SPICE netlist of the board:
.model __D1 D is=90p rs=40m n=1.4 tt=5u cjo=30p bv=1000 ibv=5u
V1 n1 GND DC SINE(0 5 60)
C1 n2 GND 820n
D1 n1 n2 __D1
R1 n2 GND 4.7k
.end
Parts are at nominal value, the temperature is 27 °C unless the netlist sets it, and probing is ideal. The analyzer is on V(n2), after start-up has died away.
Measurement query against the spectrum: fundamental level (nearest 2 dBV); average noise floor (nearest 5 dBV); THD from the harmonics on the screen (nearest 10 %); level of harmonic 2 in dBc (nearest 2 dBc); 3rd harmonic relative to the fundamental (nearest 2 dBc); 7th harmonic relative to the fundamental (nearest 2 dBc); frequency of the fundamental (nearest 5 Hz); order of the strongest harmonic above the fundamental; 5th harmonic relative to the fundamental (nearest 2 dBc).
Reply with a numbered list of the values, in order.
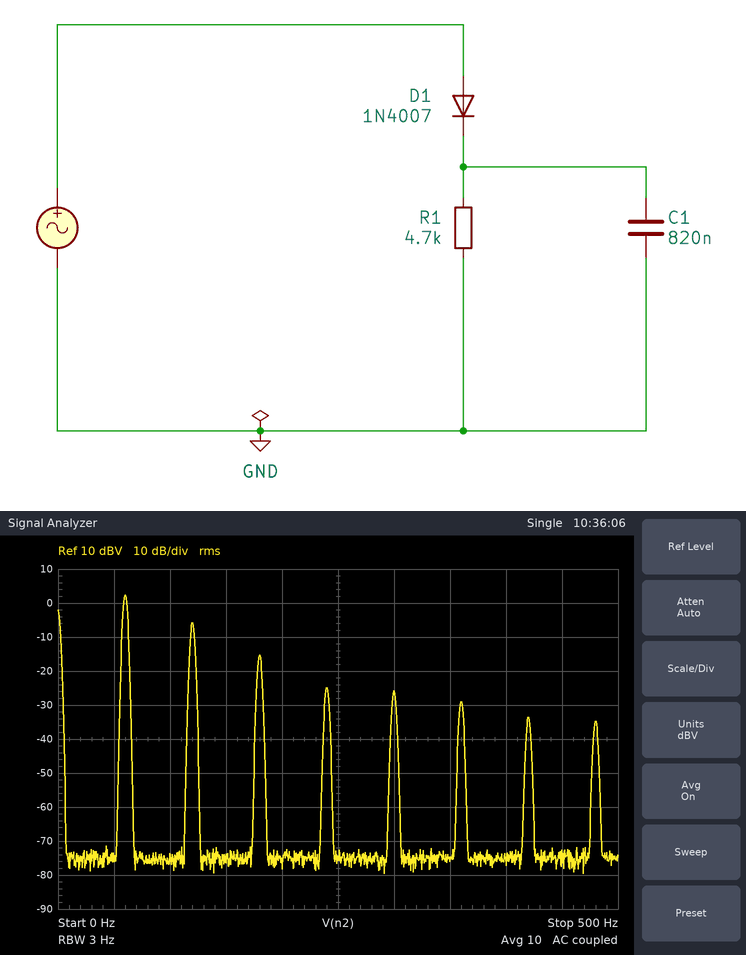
1. 2 dBV
2. -75 dBV
3. 40 %
4. -8 dBc
5. -18 dBc
6. -36 dBc
7. 60 Hz
8. 2
9. -28 dBc
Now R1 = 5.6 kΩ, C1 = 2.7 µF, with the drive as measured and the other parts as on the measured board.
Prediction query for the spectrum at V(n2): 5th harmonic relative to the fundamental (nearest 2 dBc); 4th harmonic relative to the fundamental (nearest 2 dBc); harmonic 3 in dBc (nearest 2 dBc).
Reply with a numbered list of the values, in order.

1. -24 dBc
2. -18 dBc
3. -12 dBc
